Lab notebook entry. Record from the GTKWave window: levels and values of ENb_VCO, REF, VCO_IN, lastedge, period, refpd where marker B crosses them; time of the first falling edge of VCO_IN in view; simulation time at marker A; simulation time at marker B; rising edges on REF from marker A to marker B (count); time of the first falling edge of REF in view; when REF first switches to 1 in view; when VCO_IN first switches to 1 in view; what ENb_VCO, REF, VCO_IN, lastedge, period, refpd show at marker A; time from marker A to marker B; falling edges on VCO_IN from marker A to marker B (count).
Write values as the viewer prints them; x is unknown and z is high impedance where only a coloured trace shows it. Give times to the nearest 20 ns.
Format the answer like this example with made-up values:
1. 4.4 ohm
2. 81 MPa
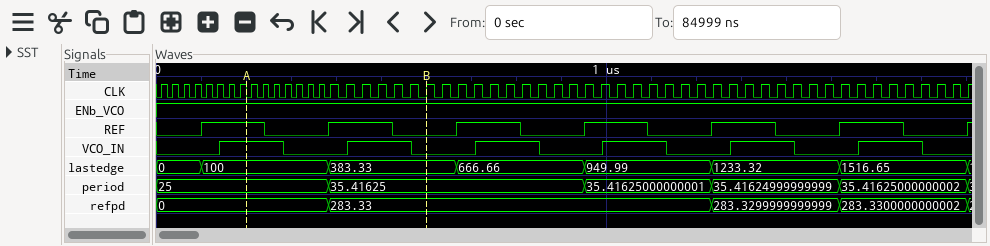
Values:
1. ENb_VCO=1, REF=0, VCO_IN=0, lastedge=383.33, period=35.41625, refpd=283.33
2. 280 ns
3. 200 ns
4. 600 ns
5. 1
6. 240 ns
7. 100 ns
8. 140 ns
9. ENb_VCO=1, REF=1, VCO_IN=1, lastedge=100, period=25, refpd=0
10. 400 ns
11. 2
